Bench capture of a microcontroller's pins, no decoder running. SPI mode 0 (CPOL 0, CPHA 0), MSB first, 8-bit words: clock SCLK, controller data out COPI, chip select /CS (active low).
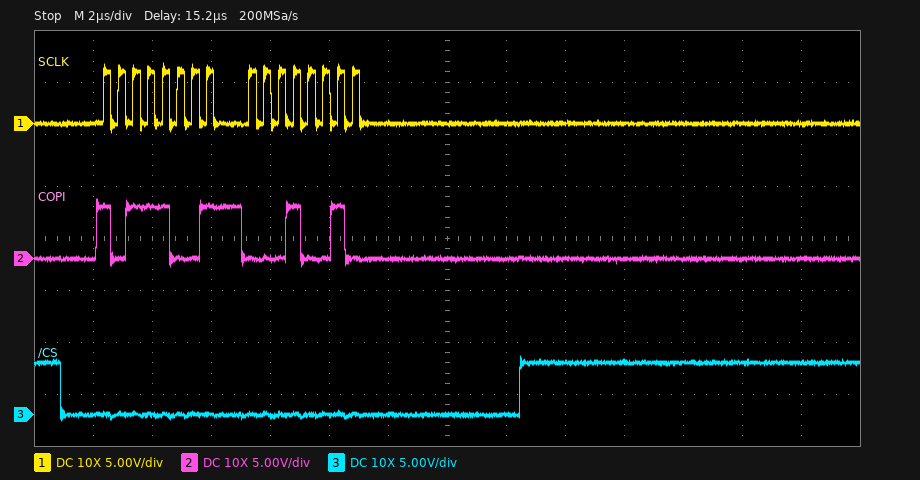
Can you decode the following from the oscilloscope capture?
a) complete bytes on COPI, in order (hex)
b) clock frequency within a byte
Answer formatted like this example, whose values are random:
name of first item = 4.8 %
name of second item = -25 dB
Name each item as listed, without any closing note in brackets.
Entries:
complete bytes on COPI, in order = B9 12
clock frequency within a byte = 2 MHz
